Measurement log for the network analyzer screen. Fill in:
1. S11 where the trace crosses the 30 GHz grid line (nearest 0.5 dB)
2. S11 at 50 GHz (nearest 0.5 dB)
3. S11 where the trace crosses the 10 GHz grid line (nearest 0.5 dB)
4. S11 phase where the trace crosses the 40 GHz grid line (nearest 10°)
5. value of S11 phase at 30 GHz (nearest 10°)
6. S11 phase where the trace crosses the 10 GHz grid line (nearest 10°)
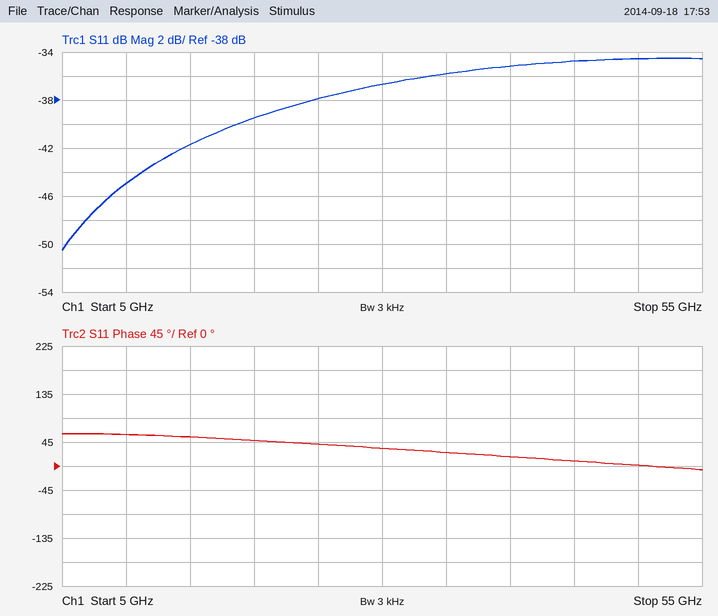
-36.5 dB
-34.5 dB
-45.0 dB
20°
30°
60°
